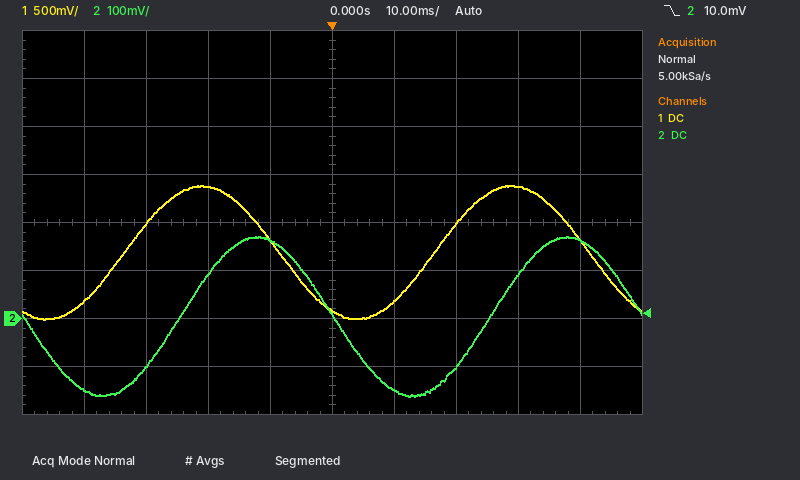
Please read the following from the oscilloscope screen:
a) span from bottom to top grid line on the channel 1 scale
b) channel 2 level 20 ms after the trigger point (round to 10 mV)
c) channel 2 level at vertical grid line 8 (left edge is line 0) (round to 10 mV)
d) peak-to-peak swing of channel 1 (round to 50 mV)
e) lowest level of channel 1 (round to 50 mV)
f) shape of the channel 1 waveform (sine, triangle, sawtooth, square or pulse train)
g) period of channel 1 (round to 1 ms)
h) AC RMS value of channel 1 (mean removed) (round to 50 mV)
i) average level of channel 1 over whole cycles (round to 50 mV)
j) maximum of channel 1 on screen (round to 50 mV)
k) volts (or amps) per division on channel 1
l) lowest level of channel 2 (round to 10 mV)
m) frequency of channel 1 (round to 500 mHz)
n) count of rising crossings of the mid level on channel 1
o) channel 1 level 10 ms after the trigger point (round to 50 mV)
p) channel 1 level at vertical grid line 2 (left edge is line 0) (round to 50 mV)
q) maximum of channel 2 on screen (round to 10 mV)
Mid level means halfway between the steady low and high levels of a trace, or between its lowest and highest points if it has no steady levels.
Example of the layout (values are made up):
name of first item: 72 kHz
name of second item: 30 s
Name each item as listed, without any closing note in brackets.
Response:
span from bottom to top grid line on the channel 1 scale: 4 V
channel 2 level 20 ms after the trigger point: -100 mV
channel 2 level at vertical grid line 8 (left edge is line 0): 90 mV
peak-to-peak swing of channel 1: 1.40 V
lowest level of channel 1: 0 mV
shape of the channel 1 waveform: sine
period of channel 1: 50 ms
AC RMS value of channel 1 (mean removed): 500 mV
average level of channel 1 over whole cycles: 700 mV
maximum of channel 1 on screen: 1.40 V
volts (or amps) per division on channel 1: 500 mV
lowest level of channel 2: -160 mV
frequency of channel 1: 20.0 Hz
count of rising crossings of the mid level on channel 1: 2
channel 1 level 10 ms after the trigger point: 200 mV
channel 1 level at vertical grid line 2 (left edge is line 0): 1.00 V
maximum of channel 2 on screen: 170 mV
